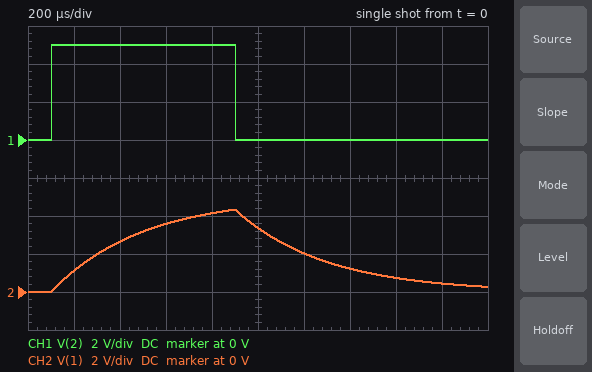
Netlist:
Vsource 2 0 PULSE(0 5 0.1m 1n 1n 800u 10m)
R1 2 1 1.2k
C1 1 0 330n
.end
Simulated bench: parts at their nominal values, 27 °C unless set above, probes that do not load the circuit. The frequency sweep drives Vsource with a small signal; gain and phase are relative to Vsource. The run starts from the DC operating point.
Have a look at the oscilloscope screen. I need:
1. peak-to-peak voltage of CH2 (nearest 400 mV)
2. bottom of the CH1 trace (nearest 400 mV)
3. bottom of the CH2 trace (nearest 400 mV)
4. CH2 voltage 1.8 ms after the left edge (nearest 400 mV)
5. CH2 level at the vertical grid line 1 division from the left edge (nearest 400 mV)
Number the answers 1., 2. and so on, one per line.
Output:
1. 4.4 V
2. 0 V
3. 0 V
4. 400 mV
5. 1.2 V
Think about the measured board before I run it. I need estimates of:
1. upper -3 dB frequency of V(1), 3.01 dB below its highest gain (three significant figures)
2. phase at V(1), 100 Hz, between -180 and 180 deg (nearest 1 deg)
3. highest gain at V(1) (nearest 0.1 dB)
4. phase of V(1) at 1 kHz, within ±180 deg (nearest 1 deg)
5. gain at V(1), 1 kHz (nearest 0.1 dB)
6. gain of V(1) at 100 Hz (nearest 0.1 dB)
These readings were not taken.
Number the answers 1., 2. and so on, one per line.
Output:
1. 402 Hz
2. -14 deg
3. 0 dB
4. -68 deg
5. -8.6 dB
6. -0.3 dB
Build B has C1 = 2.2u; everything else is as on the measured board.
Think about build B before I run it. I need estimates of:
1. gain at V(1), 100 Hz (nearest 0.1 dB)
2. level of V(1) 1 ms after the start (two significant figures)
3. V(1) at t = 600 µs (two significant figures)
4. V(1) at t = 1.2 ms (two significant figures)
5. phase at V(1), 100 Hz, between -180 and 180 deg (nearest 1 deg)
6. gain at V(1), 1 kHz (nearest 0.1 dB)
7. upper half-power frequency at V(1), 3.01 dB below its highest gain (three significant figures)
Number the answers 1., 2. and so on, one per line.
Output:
1. -5.7 dB
2. 1.3 V
3. 860 mV
4. 1.2 V
5. -59 deg
6. -24.4 dB
7. 60.3 Hz
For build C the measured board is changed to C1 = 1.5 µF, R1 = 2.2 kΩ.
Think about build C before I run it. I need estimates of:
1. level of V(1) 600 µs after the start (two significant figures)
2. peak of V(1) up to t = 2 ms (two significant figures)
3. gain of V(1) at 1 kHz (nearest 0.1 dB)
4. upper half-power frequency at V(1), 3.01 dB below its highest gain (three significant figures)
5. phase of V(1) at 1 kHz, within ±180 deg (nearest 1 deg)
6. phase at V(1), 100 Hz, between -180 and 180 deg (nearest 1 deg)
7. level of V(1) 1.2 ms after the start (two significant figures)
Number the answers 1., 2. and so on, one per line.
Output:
1. 700 mV
2. 1.1 V
3. -26.3 dB
4. 48.2 Hz
5. -87 deg
6. -64 deg
7. 980 mV
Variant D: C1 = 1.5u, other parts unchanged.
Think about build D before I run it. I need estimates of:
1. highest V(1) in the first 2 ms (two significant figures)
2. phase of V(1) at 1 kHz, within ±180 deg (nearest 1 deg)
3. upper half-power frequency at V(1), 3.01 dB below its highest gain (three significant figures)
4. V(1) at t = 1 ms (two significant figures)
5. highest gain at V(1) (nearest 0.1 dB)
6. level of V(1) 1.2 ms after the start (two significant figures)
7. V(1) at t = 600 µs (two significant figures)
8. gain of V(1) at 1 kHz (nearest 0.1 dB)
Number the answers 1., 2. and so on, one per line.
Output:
1. 1.8 V
2. -85 deg
3. 88.4 Hz
4. 1.7 V
5. 0 dB
6. 1.5 V
7. 1.2 V
8. -21.1 dB
